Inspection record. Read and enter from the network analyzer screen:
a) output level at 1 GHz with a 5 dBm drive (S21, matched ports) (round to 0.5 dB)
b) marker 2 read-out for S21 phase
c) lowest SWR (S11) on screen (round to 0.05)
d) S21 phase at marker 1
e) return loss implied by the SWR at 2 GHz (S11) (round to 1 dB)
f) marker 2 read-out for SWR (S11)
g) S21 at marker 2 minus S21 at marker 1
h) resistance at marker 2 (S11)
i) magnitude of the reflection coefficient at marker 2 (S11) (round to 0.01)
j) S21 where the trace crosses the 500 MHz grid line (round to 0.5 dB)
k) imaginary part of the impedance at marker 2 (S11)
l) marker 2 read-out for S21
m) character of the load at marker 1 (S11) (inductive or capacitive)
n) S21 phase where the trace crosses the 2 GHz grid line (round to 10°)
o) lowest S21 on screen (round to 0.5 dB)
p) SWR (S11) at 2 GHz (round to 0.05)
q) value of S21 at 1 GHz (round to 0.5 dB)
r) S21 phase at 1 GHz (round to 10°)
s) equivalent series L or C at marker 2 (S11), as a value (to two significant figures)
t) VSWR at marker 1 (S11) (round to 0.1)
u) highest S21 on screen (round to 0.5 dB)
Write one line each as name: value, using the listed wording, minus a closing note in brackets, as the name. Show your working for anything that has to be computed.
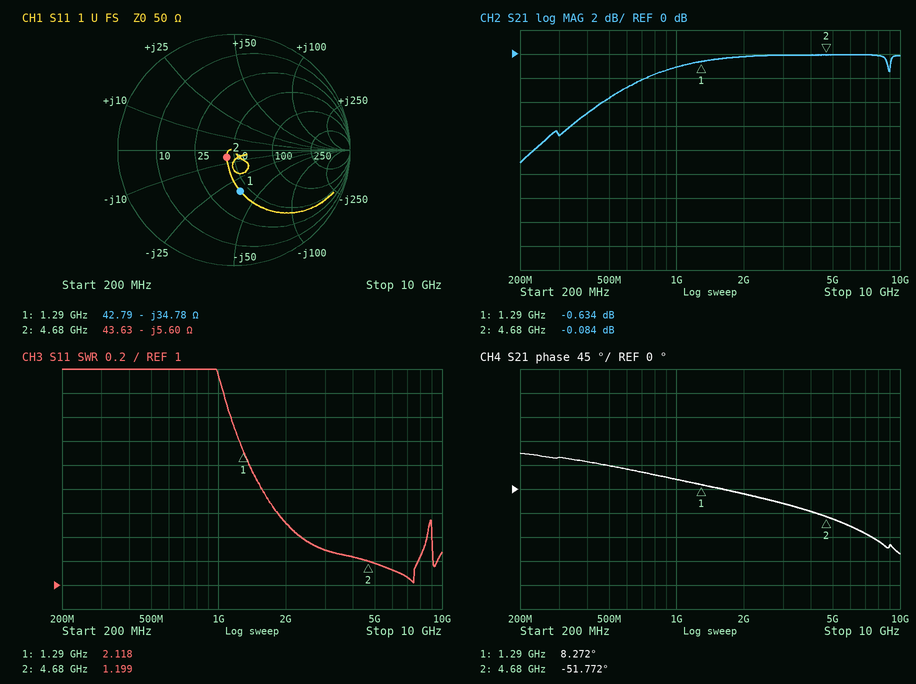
output level at 1 GHz with a 5 dBm drive (S21, matched ports): 5 dBm + (-1.0 dB) = 4.0 dBm
marker 2 read-out for S21 phase: -51.772°
lowest SWR (S11) on screen: 1.00
S21 phase at marker 1: 8.272°
return loss implied by the SWR at 2 GHz (S11): −20 log10((1.5 − 1)/(1.5 + 1)) ≈ 14 dB
marker 2 read-out for SWR: 1.199
S21 at marker 2 minus S21 at marker 1: -0.084 − (-0.634) = 0.550 dB
resistance at marker 2: 43.63 Ω
magnitude of the reflection coefficient at marker 2 (S11): 0.09
S21 where the trace crosses the 500 MHz grid line: -3.5 dB
imaginary part of the impedance at marker 2: -5.60 Ω
marker 2 read-out for S21: -0.084 dB
character of the load at marker 1 (S11): capacitive
S21 phase where the trace crosses the 2 GHz grid line: -10°
lowest S21 on screen: -9.0 dB
SWR (S11) at 2 GHz: 1.50
value of S21 at 1 GHz: -1.0 dB
S21 phase at 1 GHz: 20°
equivalent series L or C at marker 2 (S11), as a value: C = 1/(2π × 4.68 GHz × 5.6 Ω) ≈ 6.1 pF
VSWR at marker 1 (S11): 2.1
highest S21 on screen: 0.0 dB
